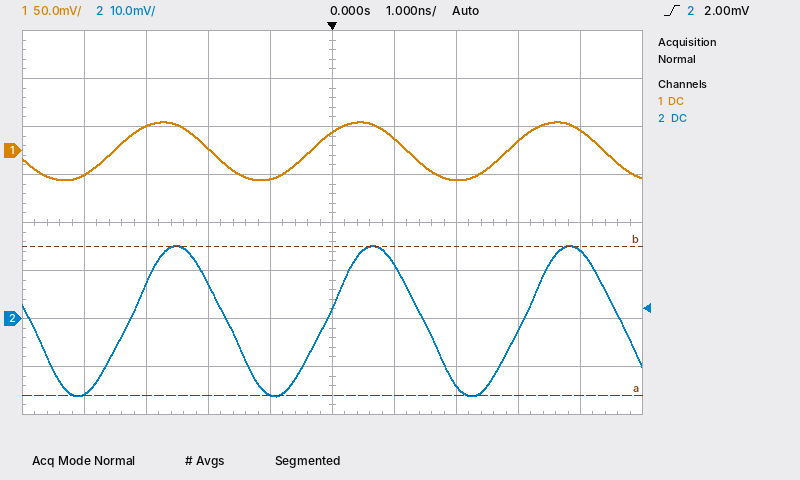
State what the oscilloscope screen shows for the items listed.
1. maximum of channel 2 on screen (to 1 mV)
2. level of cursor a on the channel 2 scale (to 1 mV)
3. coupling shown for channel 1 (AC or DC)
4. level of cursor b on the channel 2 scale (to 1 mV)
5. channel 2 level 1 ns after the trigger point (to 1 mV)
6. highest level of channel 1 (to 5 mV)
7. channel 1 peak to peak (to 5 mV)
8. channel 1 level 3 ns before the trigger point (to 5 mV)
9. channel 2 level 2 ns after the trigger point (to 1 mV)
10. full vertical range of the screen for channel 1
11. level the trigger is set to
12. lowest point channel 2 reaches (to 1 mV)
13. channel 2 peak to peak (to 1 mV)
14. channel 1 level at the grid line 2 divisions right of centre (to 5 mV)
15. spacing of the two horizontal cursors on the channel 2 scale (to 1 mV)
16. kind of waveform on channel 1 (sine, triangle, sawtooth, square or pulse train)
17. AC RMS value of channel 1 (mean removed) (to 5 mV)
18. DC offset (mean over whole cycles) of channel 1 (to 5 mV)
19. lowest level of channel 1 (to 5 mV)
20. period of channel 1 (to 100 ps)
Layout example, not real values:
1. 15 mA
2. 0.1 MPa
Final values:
1. 15 mV
2. -16 mV
3. DC
4. 15 mV
5. 11 mV
6. 30 mV
7. 60 mV
8. 25 mV
9. -14 mV
10. 400 mV
11. 2.00 mV
12. -16 mV
13. 31 mV
14. -30 mV
15. 31 mV
16. sine
17. 20 mV
18. 0 mV
19. -30 mV
20. 3.2 ns
